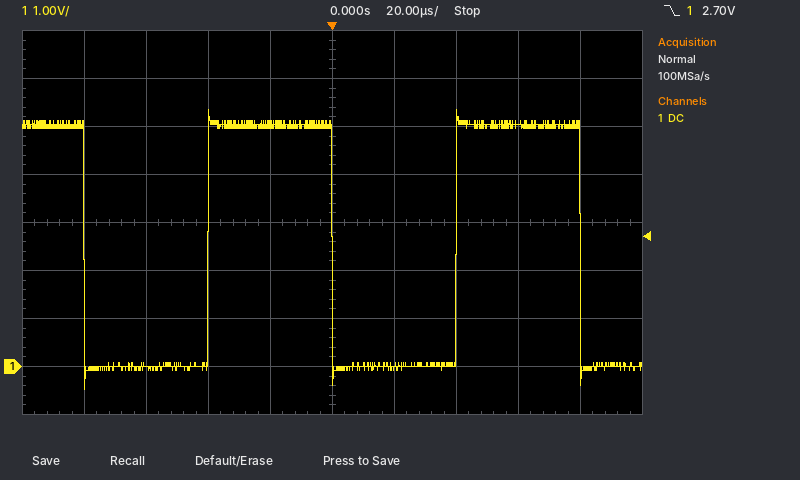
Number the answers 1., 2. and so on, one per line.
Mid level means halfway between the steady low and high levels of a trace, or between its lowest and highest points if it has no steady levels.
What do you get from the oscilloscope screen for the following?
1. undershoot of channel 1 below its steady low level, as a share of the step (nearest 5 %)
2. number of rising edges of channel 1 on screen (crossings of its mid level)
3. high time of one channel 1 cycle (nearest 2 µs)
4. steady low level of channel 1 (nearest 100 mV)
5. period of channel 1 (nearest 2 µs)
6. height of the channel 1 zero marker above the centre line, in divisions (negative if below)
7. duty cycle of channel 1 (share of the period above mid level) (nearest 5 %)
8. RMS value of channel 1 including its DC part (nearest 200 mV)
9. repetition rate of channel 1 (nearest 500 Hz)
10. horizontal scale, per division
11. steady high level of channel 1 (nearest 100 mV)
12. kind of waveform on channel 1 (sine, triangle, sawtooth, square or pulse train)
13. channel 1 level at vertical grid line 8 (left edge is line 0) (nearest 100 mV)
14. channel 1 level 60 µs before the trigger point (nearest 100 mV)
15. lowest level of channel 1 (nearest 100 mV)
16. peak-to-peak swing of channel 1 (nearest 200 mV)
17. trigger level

1. 10 %
2. 2
3. 40 µs
4. 0.0 V
5. 80 µs
6. -3.0 div
7. 50 %
8. 3.6 V
9. 12.5 kHz
10. 20 µs
11. 5.0 V
12. square
13. 5.0 V
14. 0.0 V
15. -500 mV
16. 5.8 V
17. 2.70 V
